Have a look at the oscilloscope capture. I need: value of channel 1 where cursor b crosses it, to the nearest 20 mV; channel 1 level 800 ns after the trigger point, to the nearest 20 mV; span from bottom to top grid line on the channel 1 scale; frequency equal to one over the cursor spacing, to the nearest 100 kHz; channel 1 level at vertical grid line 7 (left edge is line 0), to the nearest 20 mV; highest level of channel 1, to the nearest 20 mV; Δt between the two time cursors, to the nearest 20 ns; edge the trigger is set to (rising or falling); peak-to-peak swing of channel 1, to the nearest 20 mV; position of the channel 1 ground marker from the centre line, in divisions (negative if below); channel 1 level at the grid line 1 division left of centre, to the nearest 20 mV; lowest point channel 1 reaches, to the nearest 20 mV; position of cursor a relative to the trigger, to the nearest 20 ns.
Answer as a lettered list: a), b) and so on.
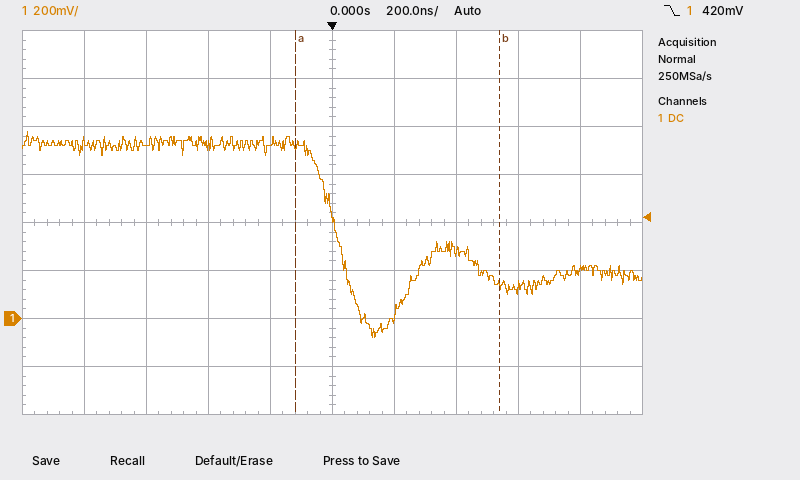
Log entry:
a) 140 mV
b) 200 mV
c) 1.6 V
d) 1.5 MHz
e) 280 mV
f) 780 mV
g) 660 ns
h) falling
i) 860 mV
j) -2.0 div
k) 740 mV
l) -80 mV
m) -120 ns
